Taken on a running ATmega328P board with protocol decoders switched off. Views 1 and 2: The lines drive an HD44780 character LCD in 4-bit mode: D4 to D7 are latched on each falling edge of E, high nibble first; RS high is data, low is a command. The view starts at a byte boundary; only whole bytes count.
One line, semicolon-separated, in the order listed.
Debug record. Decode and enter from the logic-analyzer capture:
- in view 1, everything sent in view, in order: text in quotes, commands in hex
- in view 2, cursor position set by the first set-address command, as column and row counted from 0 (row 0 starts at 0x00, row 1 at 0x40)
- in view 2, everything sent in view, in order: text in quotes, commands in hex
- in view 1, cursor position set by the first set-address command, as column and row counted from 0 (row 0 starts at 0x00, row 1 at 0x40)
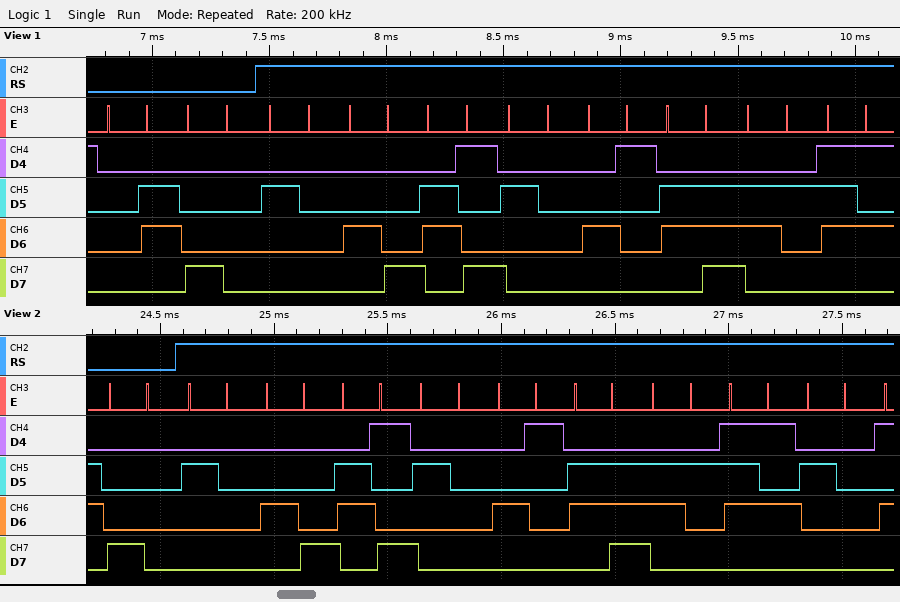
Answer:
0x06 0x80 " Hi Anbu"; column 0, row 0; 0x80 " Hi Anbu "; column 0, row 0
